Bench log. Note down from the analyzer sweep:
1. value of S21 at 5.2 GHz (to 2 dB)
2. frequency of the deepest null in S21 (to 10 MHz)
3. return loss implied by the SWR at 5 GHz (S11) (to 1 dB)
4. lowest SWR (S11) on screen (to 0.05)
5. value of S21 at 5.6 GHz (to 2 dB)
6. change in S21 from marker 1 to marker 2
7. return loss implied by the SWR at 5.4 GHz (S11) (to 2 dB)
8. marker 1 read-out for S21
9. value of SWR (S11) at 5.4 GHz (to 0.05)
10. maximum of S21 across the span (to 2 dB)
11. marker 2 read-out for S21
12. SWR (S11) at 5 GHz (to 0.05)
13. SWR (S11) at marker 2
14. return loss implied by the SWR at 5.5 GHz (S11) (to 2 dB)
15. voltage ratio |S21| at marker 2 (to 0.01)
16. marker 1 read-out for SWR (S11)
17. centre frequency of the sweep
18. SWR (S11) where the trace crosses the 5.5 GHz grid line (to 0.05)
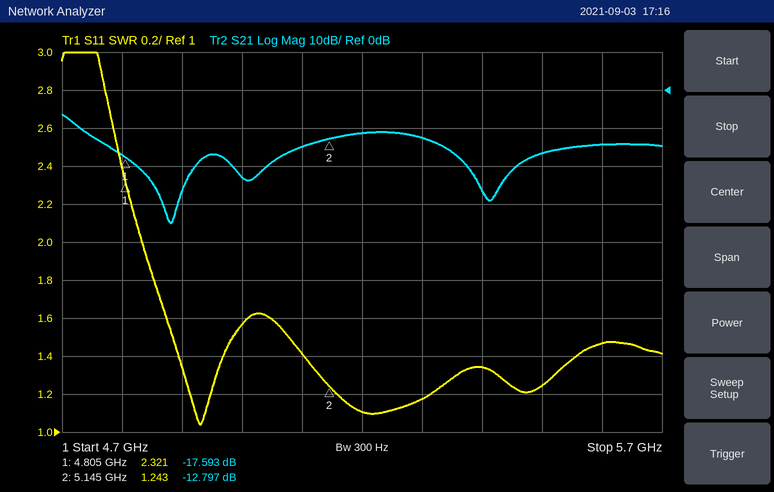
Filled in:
-12 dB
4.88 GHz
13 dB
1.05
-14 dB
4.796 dB
16 dB
-17.593 dB
1.35
-6 dB
-12.797 dB
1.55
1.243
20 dB
0.23
2.321
5.2 GHz
1.25
